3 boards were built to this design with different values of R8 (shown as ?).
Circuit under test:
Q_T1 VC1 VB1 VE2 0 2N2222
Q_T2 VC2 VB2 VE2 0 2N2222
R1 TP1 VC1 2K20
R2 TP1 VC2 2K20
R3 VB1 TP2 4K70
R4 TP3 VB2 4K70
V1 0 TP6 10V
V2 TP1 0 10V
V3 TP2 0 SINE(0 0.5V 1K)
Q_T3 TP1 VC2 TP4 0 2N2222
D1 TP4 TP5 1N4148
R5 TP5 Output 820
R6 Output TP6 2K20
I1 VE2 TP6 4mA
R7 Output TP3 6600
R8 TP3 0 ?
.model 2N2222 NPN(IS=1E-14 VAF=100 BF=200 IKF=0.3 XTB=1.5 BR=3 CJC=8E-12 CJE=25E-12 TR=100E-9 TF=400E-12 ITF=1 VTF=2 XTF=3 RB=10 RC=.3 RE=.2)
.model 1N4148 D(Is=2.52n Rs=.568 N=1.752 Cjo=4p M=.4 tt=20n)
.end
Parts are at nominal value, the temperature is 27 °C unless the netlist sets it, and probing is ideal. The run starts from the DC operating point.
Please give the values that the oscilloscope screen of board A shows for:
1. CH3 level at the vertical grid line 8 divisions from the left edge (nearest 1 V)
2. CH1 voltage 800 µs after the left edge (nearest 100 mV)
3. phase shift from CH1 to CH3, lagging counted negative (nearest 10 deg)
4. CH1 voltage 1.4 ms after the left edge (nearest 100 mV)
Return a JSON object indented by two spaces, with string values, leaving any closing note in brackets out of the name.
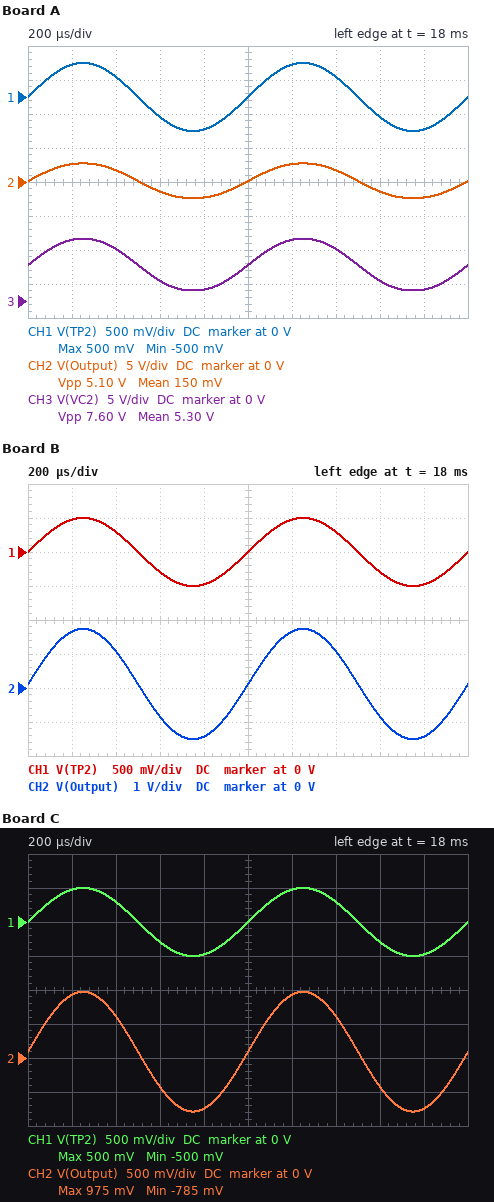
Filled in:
{
  "CH3 level at the vertical grid line 8 divisions from the left edge": "3 V",
  "CH1 voltage 800 µs after the left edge": "-500 mV",
  "phase shift from CH1 to CH3, lagging counted negative": "0 deg",
  "CH1 voltage 1.4 ms after the left edge": "300 mV"
}
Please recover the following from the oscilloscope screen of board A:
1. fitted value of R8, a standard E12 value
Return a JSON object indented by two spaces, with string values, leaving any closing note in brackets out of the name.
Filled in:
{
  "fitted value of R8, a standard E12 value": "1 kΩ"
}
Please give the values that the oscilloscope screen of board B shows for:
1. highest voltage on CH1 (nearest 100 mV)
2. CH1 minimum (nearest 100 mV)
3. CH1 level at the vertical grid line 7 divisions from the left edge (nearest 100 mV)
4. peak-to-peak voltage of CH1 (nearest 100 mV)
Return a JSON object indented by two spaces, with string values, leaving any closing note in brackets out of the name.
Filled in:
{
  "highest voltage on CH1": "500 mV",
  "CH1 minimum": "-500 mV",
  "CH1 level at the vertical grid line 7 divisions from the left edge": "300 mV",
  "peak-to-peak voltage of CH1": "1.0 V"
}
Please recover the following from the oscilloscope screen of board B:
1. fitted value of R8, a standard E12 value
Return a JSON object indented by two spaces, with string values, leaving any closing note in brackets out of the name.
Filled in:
{
  "fitted value of R8, a standard E12 value": "2.2 kΩ"
}
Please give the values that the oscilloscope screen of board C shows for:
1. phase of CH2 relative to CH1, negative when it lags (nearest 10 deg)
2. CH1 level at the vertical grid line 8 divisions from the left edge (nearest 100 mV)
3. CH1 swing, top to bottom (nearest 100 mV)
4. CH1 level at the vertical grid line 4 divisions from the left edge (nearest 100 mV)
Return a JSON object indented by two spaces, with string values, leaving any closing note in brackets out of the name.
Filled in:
{
  "phase of CH2 relative to CH1, negative when it lags": "0 deg",
  "CH1 level at the vertical grid line 8 divisions from the left edge": "-300 mV",
  "CH1 swing, top to bottom": "1.0 V",
  "CH1 level at the vertical grid line 4 divisions from the left edge": "-500 mV"
}
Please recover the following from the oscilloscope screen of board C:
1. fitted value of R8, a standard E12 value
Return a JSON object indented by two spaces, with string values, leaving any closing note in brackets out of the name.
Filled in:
{
  "fitted value of R8, a standard E12 value": "6.8 kΩ"
}
